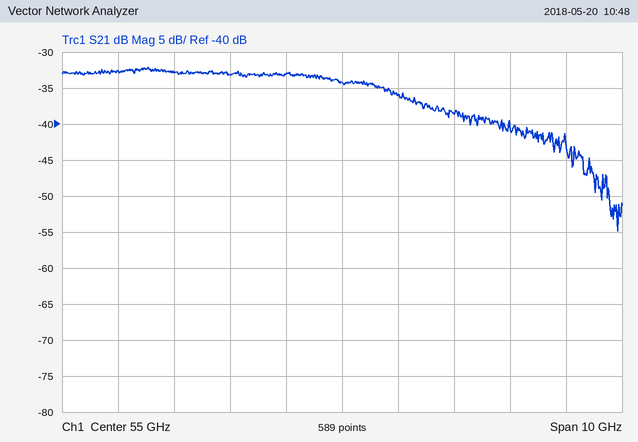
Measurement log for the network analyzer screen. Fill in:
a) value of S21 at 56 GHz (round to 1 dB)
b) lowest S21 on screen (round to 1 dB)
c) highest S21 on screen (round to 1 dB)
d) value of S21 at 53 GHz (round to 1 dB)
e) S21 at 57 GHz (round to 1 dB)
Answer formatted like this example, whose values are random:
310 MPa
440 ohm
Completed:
-36 dB
-55 dB
-32 dB
-33 dB
-39 dB
